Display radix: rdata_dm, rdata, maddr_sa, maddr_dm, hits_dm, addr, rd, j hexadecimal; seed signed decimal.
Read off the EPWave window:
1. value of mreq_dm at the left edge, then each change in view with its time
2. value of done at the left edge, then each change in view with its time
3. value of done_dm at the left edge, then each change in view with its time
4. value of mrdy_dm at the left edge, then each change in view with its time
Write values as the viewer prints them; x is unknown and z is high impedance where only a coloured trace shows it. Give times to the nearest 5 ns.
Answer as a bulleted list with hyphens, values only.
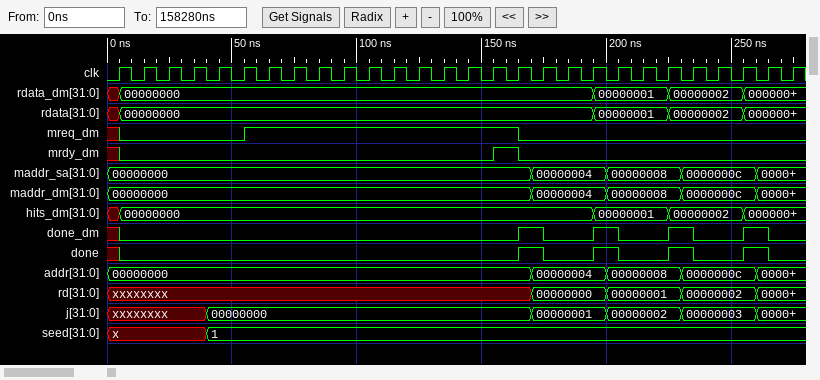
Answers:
- x, 0 at 5 ns, 1 at 55 ns, 0 at 165 ns
- x, 0 at 5 ns, 1 at 165 ns, 0 at 175 ns, 1 at 195 ns, 0 at 205 ns, 1 at 225 ns, 0 at 235 ns, 1 at 255 ns, 0 at 265 ns
- x, 0 at 5 ns, 1 at 165 ns, 0 at 175 ns, 1 at 195 ns, 0 at 205 ns, 1 at 225 ns, 0 at 235 ns, 1 at 255 ns, 0 at 265 ns
- x, 0 at 5 ns, 1 at 155 ns, 0 at 165 ns
